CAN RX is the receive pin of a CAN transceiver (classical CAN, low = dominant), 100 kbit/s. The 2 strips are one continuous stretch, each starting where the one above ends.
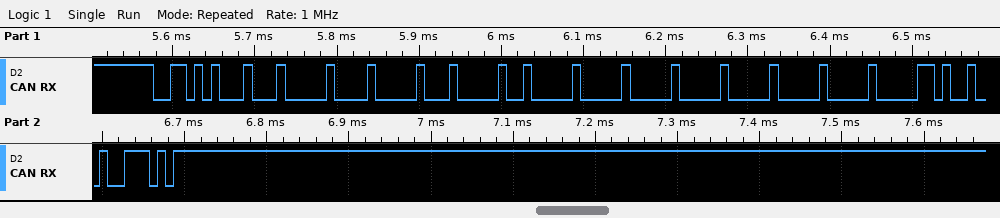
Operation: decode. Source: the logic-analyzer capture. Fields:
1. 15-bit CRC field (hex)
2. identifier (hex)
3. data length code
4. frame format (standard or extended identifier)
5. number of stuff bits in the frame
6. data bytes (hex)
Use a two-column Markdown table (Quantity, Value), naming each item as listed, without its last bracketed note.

| Quantity | Value |
|---|---|
| 15-bit CRC field | 0x524E |
| identifier | 0x351 |
| data length code | 8 |
| frame format | standard |
| number of stuff bits in the frame | 11 |
| data bytes | 02 01 01 00 00 00 00 00 |
